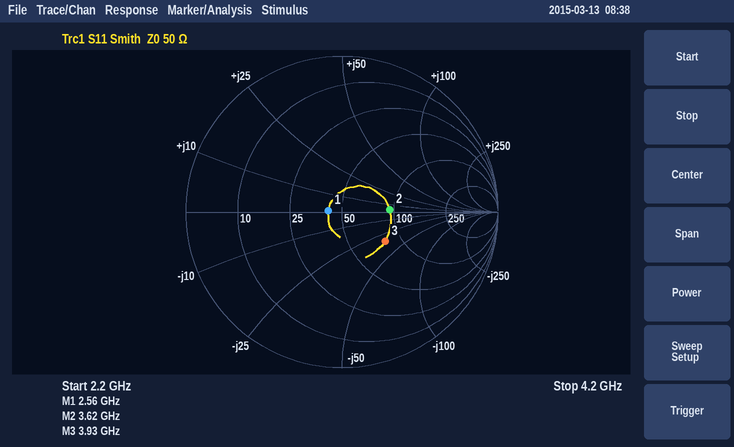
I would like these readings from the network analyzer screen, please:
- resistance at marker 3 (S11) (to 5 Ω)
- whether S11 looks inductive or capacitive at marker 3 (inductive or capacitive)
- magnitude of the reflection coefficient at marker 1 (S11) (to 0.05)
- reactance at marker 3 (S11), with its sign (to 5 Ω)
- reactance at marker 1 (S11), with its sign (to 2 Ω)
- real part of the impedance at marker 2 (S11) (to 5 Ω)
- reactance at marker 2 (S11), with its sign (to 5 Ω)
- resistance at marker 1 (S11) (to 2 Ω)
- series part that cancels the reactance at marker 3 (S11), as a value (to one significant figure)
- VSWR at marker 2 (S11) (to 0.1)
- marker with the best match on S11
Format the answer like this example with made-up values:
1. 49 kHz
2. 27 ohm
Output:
1. 80 Ω
2. capacitive
3. 0.10
4. -35 Ω
5. 0 Ω
6. 95 Ω
7. +5 Ω
8. 42 Ω
9. 1 nH
10. 1.9
11. marker 1
